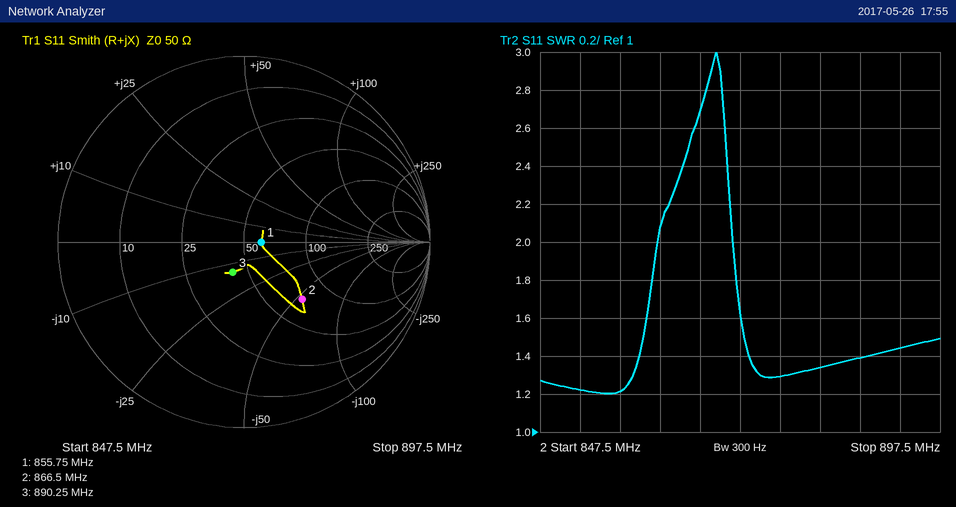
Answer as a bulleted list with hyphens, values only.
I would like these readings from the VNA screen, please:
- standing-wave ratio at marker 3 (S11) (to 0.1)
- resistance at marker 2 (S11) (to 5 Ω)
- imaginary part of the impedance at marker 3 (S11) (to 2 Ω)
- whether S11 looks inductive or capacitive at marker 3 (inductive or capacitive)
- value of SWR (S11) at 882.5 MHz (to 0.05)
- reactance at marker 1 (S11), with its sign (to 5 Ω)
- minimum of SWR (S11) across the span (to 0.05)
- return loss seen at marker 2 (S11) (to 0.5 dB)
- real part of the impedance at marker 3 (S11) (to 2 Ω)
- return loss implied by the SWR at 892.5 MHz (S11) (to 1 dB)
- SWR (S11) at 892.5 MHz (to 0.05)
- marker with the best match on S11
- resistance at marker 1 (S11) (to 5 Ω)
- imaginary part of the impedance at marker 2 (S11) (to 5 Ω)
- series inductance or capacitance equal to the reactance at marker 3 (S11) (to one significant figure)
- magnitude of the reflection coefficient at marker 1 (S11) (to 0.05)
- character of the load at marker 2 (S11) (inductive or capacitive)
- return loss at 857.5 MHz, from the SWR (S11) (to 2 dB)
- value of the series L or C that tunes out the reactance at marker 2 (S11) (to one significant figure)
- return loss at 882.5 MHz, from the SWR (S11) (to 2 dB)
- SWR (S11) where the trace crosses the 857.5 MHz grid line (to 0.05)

- 1.4
- 70 Ω
- -14 Ω
- capacitive
- 1.35
- 0 Ω
- 1.20
- 7.0 dB
- 42 Ω
- 15 dB
- 1.45
- marker 1
- 60 Ω
- -55 Ω
- 10 pF
- 0.10
- capacitive
- 20 dB
- 10 nH
- 16 dB
- 1.20
